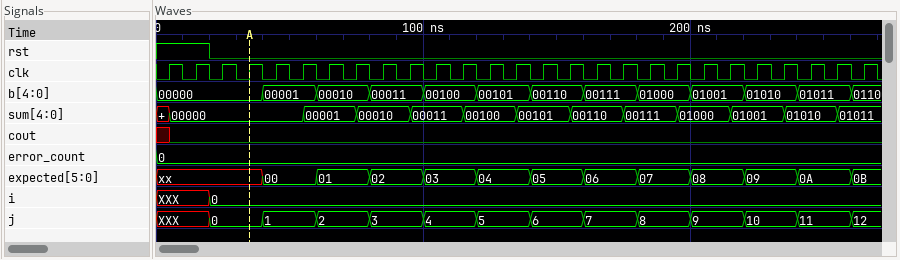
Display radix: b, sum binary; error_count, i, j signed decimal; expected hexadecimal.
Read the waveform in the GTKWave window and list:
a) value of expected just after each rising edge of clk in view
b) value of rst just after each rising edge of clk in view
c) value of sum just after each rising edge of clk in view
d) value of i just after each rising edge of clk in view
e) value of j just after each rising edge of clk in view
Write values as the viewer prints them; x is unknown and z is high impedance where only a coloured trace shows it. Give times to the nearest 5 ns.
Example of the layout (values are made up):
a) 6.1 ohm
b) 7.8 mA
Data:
a) xx, xx, xx, xx, 00, 00, 01, 01, 02, 02, 03, 03, 04, 04, 05, 05, 06, 06, 07, 07, 08, 08, 09, 09, 0A, 0A, 0B
b) 1 1 0 0 0 0 0 0 0 0 0 0 0 0 0 0 0 0 0 0 0 0 0 0 0 0 0
c) 00000, 00000, 00000, 00000, 00000, 00001, 00001, 00010, 00010, 00011, 00011, 00100, 00100, 00101, 00101, 00110, 00110, 00111, 00111, 01000, 01000, 01001, 01001, 01010, 01010, 01011, 01011
d) XXX, XXX, 0, 0, 0, 0, 0, 0, 0, 0, 0, 0, 0, 0, 0, 0, 0, 0, 0, 0, 0, 0, 0, 0, 0, 0, 0
e) XXX, XXX, 0, 0, 1, 1, 2, 2, 3, 3, 4, 4, 5, 5, 6, 6, 7, 7, 8, 8, 9, 9, 10, 10, 11, 11, 12
